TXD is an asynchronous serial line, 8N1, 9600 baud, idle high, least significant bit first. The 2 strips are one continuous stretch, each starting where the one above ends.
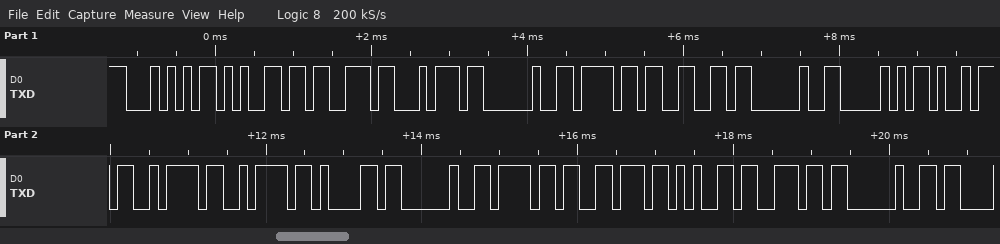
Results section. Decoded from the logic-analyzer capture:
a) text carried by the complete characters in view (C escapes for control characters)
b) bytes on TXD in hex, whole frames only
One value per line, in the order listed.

"Test of Pizza oven "
54 65 73 74 20 6F 66 20 50 69 7A 7A 61 20 6F 76 65 6E 20
